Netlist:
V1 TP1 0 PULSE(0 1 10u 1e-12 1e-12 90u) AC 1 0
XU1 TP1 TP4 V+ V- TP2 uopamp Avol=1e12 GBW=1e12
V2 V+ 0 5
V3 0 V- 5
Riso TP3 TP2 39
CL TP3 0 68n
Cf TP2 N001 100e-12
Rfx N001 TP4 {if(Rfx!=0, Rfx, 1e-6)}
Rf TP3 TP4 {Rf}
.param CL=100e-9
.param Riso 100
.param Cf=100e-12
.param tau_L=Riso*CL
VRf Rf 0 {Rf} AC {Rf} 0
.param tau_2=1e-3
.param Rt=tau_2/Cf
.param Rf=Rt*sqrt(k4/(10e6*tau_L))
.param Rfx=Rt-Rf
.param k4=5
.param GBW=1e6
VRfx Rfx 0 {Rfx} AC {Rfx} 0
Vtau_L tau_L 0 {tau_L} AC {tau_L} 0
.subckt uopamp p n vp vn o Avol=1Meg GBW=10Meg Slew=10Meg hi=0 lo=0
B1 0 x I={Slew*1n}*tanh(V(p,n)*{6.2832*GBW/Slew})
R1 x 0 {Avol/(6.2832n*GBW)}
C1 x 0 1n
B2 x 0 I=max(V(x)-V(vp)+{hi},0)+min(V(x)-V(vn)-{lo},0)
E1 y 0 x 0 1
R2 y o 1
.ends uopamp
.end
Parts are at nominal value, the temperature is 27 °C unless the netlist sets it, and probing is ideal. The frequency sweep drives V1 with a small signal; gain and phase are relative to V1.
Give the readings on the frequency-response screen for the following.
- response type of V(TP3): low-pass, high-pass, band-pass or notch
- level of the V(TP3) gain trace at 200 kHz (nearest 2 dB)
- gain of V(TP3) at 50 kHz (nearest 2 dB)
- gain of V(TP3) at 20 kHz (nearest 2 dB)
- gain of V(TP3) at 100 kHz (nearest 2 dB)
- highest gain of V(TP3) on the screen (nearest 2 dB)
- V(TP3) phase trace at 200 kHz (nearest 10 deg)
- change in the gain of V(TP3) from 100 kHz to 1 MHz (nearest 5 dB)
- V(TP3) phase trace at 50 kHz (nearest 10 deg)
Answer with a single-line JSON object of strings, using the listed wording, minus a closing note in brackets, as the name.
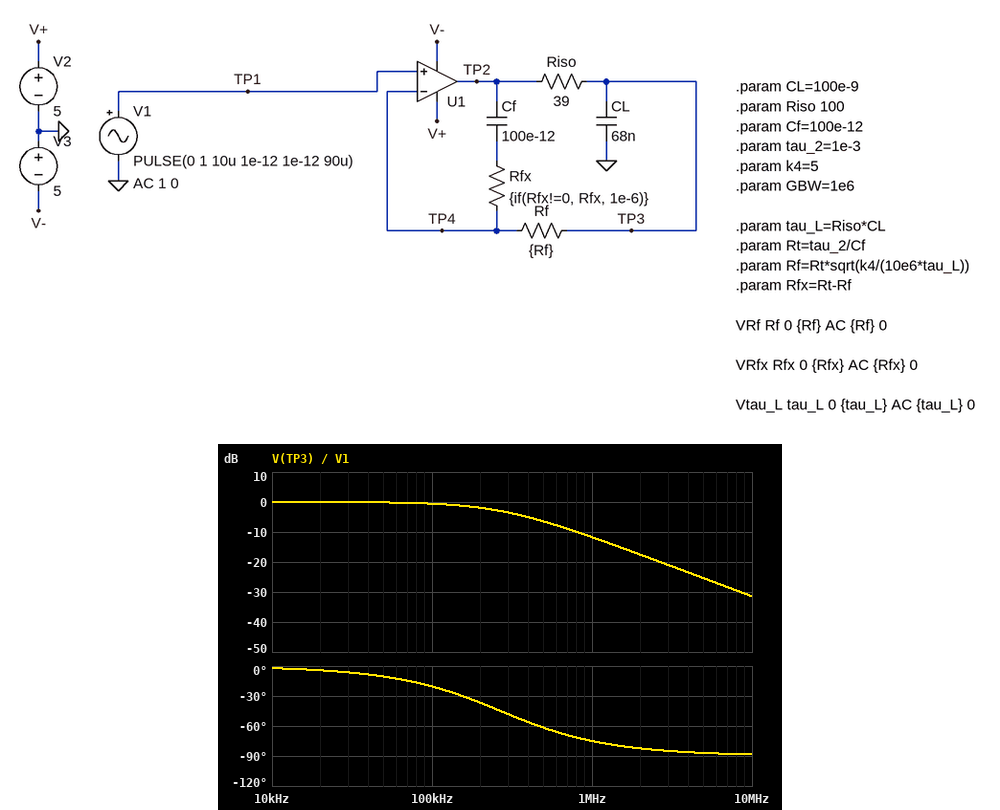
{"response type of V(TP3): low-pass, high-pass, band-pass or notch": "low-pass", "level of the V(TP3) gain trace at 200 kHz": "-2 dB", "gain of V(TP3) at 50 kHz": "0 dB", "gain of V(TP3) at 20 kHz": "0 dB", "gain of V(TP3) at 100 kHz": "0 dB", "highest gain of V(TP3) on the screen": "0 dB", "V(TP3) phase trace at 200 kHz": "-40 deg", "change in the gain of V(TP3) from 100 kHz to 1 MHz": "-10 dB", "V(TP3) phase trace at 50 kHz": "-10 deg"}
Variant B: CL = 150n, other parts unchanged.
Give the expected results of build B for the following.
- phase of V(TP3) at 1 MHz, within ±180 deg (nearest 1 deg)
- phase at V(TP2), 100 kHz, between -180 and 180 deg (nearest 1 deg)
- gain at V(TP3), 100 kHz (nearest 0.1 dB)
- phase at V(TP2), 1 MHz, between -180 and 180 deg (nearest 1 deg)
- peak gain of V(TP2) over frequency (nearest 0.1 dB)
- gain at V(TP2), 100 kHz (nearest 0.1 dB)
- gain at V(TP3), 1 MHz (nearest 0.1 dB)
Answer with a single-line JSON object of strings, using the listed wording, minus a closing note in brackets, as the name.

{"phase of V(TP3) at 1 MHz, within ±180 deg": "-83 deg", "phase at V(TP2), 100 kHz, between -180 and 180 deg": "35 deg", "gain at V(TP3), 100 kHz": "-2.2 dB", "phase at V(TP2), 1 MHz, between -180 and 180 deg": "5 deg", "peak gain of V(TP2) over frequency": "13.0 dB", "gain at V(TP2), 100 kHz": "9.4 dB", "gain at V(TP3), 1 MHz": "-18.4 dB"}
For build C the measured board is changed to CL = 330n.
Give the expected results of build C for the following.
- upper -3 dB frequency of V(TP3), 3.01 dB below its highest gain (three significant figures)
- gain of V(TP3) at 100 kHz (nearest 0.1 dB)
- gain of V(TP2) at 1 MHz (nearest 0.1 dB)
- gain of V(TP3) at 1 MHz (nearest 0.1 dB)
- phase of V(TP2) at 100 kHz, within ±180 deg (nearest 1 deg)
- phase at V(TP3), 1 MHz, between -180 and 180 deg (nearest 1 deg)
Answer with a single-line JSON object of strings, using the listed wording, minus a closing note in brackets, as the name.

{"upper -3 dB frequency of V(TP3), 3.01 dB below its highest gain": "55.2 kHz", "gain of V(TP3) at 100 kHz": "-6.3 dB", "gain of V(TP2) at 1 MHz": "13.0 dB", "gain of V(TP3) at 1 MHz": "-25.2 dB", "phase of V(TP2) at 100 kHz, within ±180 deg": "22 deg", "phase at V(TP3), 1 MHz, between -180 and 180 deg": "-87 deg"}
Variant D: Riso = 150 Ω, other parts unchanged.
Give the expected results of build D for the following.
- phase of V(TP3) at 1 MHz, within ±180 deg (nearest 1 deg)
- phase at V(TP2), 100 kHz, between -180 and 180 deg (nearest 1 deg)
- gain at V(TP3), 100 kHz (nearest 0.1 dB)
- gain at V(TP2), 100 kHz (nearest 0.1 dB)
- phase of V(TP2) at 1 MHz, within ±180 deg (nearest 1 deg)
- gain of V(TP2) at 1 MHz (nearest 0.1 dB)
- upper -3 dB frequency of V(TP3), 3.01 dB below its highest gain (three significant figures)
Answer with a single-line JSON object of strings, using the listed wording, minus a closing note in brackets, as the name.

{"phase of V(TP3) at 1 MHz, within ±180 deg": "-86 deg", "phase at V(TP2), 100 kHz, between -180 and 180 deg": "26 deg", "gain at V(TP3), 100 kHz": "-4.8 dB", "gain at V(TP2), 100 kHz": "11.4 dB", "phase of V(TP2) at 1 MHz, within ±180 deg": "3 deg", "gain of V(TP2) at 1 MHz": "13.0 dB", "upper -3 dB frequency of V(TP3), 3.01 dB below its highest gain": "69.6 kHz"}
